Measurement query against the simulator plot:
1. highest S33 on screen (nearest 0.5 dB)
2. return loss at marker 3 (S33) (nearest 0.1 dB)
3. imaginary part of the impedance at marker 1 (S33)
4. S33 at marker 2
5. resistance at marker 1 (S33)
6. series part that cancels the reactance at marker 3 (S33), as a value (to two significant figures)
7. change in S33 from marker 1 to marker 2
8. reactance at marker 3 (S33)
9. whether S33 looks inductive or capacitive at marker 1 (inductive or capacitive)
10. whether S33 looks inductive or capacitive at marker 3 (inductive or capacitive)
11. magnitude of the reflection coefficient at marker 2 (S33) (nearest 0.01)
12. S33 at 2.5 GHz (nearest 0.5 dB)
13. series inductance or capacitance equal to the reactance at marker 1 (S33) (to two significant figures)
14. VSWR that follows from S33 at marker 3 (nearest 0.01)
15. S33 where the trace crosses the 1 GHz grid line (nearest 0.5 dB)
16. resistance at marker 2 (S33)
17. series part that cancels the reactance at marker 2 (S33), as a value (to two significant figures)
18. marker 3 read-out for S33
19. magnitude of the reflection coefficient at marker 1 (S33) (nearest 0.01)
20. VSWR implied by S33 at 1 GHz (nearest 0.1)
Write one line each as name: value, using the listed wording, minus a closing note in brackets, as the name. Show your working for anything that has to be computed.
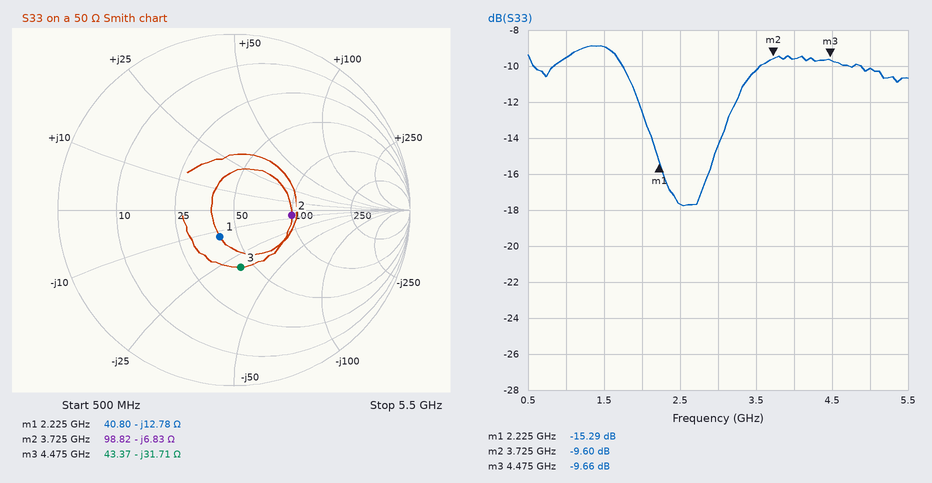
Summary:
highest S33 on screen: -9.0 dB
return loss at marker 3 (S33): 9.7 dB
imaginary part of the impedance at marker 1: -12.78 Ω
S33 at marker 2: -9.60 dB
resistance at marker 1: 40.80 Ω
series part that cancels the reactance at marker 3 (S33), as a value: L = 31.71 Ω/(2π × 4.475 GHz) ≈ 1.1 nH
change in S33 from marker 1 to marker 2: -9.6 − (-15.29) = 5.69 dB
reactance at marker 3: -31.71 Ω
whether S33 looks inductive or capacitive at marker 1: capacitive
whether S33 looks inductive or capacitive at marker 3: capacitive
magnitude of the reflection coefficient at marker 2 (S33): 0.33
S33 at 2.5 GHz: -17.5 dB
series inductance or capacitance equal to the reactance at marker 1 (S33): C = 1/(2π × 2.225 GHz × 12.78 Ω) ≈ 5.6 pF
VSWR that follows from S33 at marker 3: (1 + 0.3289)/(1 − 0.3289) ≈ 1.98
S33 where the trace crosses the 1 GHz grid line: -9.5 dB
resistance at marker 2: 98.82 Ω
series part that cancels the reactance at marker 2 (S33), as a value: L = 6.83 Ω/(2π × 3.725 GHz) ≈ 292 pH, so 290 pH to two significant figures
marker 3 read-out for S33: -9.66 dB
magnitude of the reflection coefficient at marker 1 (S33): 10^(-15.29/20) ≈ 0.17
VSWR implied by S33 at 1 GHz: |Γ| = 10^(-9.5/20) = 0.3350; VSWR = (1 + 0.3350)/(1 − 0.3350) ≈ 2.0
